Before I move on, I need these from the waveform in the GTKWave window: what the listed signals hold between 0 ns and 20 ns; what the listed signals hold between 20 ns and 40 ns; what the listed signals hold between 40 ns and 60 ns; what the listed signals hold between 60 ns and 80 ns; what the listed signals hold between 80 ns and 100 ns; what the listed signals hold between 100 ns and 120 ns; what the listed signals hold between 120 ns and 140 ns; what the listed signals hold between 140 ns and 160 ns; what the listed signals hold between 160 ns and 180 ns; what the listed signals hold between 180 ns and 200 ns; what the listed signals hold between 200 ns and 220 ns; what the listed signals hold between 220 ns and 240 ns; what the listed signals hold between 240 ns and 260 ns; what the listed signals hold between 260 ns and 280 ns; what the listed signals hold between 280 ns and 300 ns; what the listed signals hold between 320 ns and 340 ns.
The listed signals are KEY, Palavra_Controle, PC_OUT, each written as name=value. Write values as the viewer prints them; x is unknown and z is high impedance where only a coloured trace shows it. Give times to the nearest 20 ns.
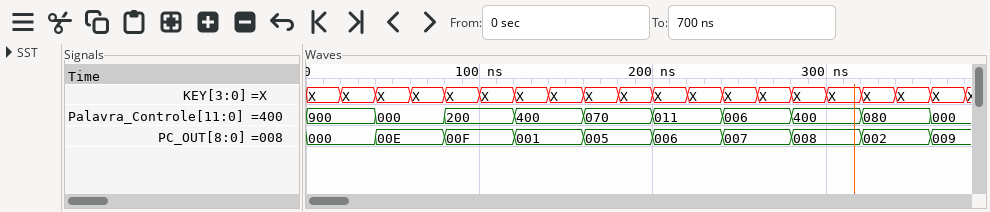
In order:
KEY=X, Palavra_Controle=900, PC_OUT=000
KEY=X, Palavra_Controle=900, PC_OUT=000
KEY=X, Palavra_Controle=000, PC_OUT=00E
KEY=X, Palavra_Controle=000, PC_OUT=00E
KEY=X, Palavra_Controle=200, PC_OUT=00F
KEY=X, Palavra_Controle=200, PC_OUT=00F
KEY=X, Palavra_Controle=400, PC_OUT=001
KEY=X, Palavra_Controle=400, PC_OUT=001
KEY=X, Palavra_Controle=070, PC_OUT=005
KEY=X, Palavra_Controle=070, PC_OUT=005
KEY=X, Palavra_Controle=011, PC_OUT=006
KEY=X, Palavra_Controle=011, PC_OUT=006
KEY=X, Palavra_Controle=006, PC_OUT=007
KEY=X, Palavra_Controle=006, PC_OUT=007
KEY=X, Palavra_Controle=400, PC_OUT=008
KEY=X, Palavra_Controle=080, PC_OUT=002
